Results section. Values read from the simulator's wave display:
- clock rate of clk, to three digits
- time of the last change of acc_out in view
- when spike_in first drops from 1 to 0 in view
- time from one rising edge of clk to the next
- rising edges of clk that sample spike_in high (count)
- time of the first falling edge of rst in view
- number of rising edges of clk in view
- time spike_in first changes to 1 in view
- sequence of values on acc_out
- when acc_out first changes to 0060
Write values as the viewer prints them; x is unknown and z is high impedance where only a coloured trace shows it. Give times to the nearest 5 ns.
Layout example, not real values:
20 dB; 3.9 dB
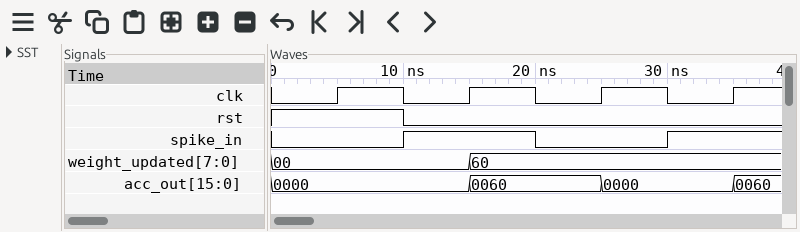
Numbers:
100 MHz; 35 ns; 20 ns; 10 ns; 2; 10 ns; 4; 10 ns; 0000, 0060, 0000, 0060; 15 ns
